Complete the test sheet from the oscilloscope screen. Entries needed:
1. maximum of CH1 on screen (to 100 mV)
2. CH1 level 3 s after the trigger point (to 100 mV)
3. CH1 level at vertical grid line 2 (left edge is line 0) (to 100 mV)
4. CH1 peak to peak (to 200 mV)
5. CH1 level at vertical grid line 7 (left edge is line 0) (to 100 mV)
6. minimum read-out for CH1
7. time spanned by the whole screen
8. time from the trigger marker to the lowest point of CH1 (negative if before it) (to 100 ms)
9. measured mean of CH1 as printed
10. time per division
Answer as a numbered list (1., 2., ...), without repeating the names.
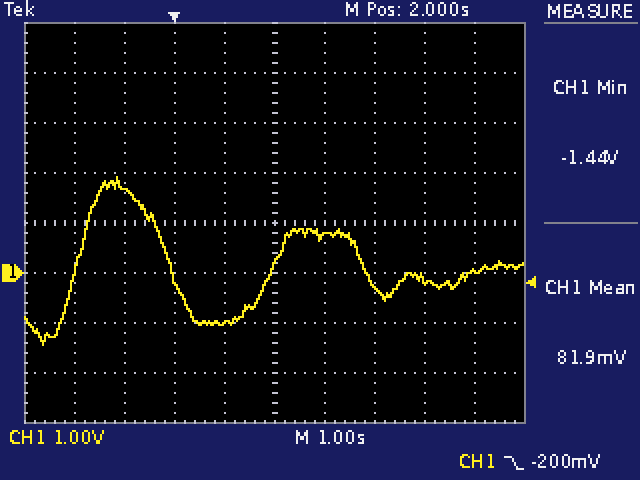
1. 1.9 V
2. 700 mV
3. 1.7 V
4. 3.4 V
5. -300 mV
6. -1.44 V
7. 10 s
8. -2.6 s
9. 81.9 mV
10. 1 s
